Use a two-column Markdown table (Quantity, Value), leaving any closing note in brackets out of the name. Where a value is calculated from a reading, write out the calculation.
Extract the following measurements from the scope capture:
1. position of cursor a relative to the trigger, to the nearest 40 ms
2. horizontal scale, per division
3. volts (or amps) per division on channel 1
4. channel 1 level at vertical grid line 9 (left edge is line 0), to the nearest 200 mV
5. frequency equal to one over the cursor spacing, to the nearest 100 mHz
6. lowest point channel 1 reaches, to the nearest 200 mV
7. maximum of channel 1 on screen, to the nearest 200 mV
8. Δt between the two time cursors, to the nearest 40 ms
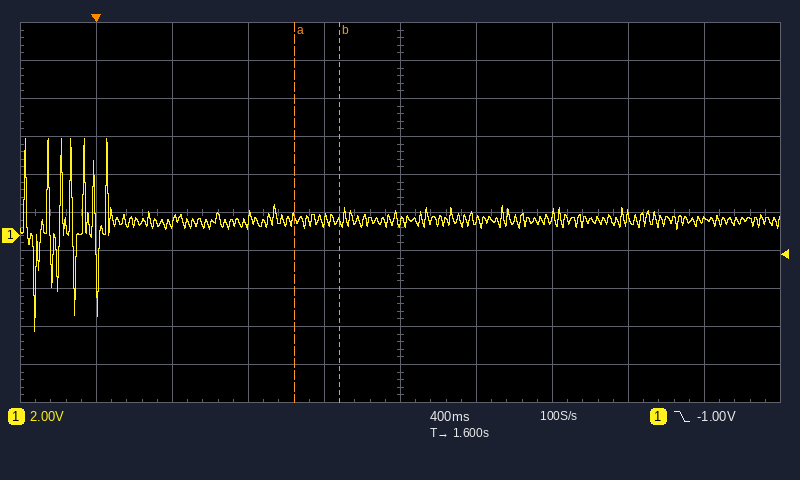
| Quantity | Value |
|---|---|
| position of cursor a relative to the trigger, to the nearest 40 ms | +1.04 s |
| horizontal scale, per division | 400 ms |
| volts (or amps) per division on channel 1 | 2 V |
| channel 1 level at vertical grid line 9 (left edge is line 0), to the nearest 200 mV | 800 mV |
| frequency equal to one over the cursor spacing, to the nearest 100 mHz | 1 / 240 ms ≈ 4.2 Hz |
| lowest point channel 1 reaches, to the nearest 200 mV | -5.0 V |
| maximum of channel 1 on screen, to the nearest 200 mV | 5.0 V |
| Δt between the two time cursors, to the nearest 40 ms | 240 ms |
